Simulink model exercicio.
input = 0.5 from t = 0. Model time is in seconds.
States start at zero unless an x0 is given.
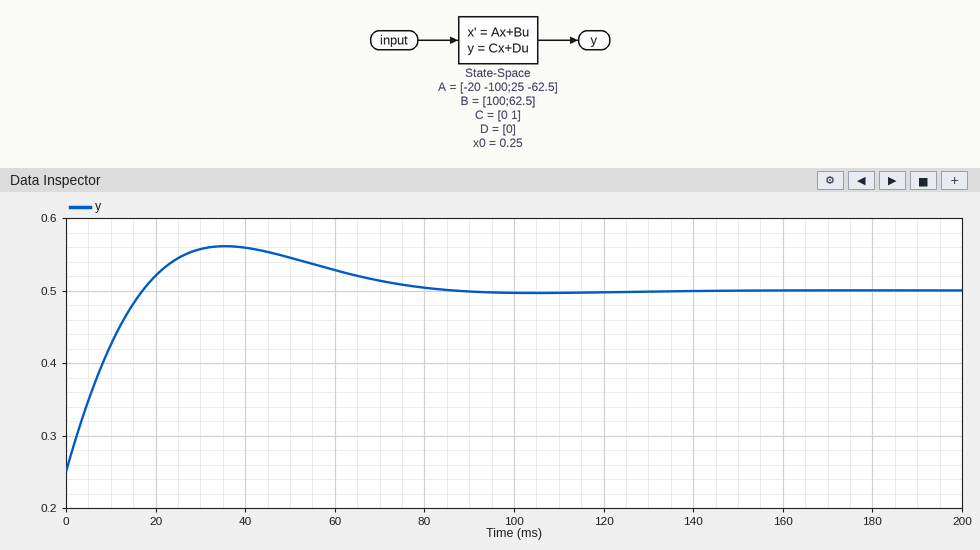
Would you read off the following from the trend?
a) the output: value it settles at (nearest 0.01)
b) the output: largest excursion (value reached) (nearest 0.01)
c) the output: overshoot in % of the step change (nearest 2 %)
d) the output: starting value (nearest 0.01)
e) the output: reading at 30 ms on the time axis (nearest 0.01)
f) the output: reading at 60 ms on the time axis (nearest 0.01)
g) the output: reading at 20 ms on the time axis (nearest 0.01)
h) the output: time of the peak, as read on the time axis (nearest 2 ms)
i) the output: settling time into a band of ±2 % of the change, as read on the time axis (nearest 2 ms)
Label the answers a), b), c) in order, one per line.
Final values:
a) 0.50
b) 0.56
c) 24 %
d) 0.25
e) 0.56
f) 0.53
g) 0.52
h) 36 ms
i) 78 ms
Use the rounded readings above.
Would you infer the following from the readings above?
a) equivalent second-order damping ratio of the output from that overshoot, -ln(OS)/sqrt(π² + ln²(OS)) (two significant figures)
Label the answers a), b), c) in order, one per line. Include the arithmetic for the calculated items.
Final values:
a) ln(0.24) = -1.427; 1.427 / sqrt(9.870 + 2.037) = 0.41
